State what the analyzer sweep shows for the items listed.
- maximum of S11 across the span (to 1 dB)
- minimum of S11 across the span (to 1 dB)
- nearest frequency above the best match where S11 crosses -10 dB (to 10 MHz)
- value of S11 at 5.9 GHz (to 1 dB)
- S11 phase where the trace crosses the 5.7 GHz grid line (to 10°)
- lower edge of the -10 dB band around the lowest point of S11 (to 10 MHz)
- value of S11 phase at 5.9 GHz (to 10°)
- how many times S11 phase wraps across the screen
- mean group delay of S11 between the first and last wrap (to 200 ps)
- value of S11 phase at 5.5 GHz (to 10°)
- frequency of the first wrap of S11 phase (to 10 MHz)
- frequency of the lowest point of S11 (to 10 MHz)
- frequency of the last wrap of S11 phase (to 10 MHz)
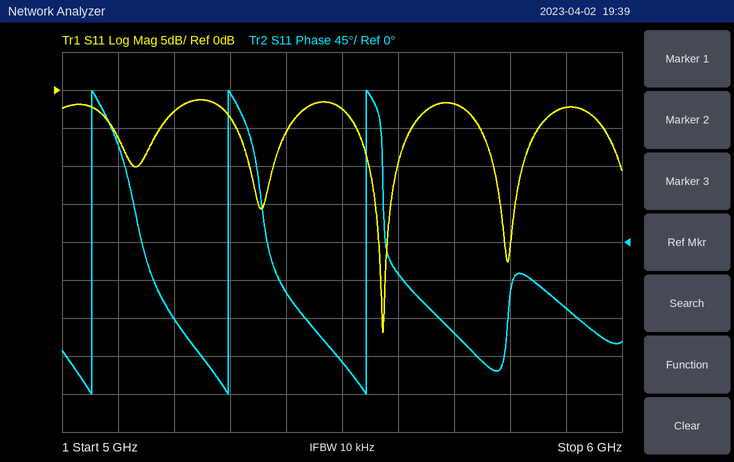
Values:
-1 dB
-32 dB
5.60 GHz
-2 dB
-110°
5.55 GHz
-80°
3
4.0 ns
-140°
5.05 GHz
5.57 GHz
5.54 GHz
